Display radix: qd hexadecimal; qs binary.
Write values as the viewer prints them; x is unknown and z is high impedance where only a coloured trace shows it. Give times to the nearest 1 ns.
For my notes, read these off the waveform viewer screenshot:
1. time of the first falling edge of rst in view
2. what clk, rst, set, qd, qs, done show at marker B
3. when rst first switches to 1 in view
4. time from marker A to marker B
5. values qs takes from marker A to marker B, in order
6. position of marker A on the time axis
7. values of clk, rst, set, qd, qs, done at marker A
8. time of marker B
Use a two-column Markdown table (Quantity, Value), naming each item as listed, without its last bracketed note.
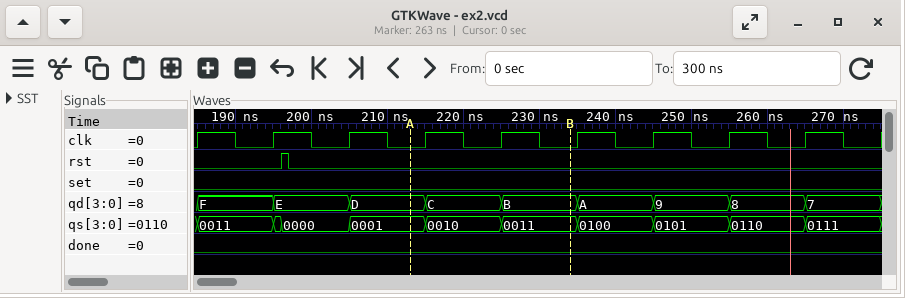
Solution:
| Quantity | Value |
|---|---|
| time of the first falling edge of rst in view | 197 ns |
| what clk, rst, set, qd, qs, done show at marker B | clk=0, rst=0, set=0, qd=B, qs=0011, done=0 |
| when rst first switches to 1 in view | 196 ns |
| time from marker A to marker B | 21 ns |
| values qs takes from marker A to marker B, in order | 0001, 0010, 0011 |
| position of marker A on the time axis | 213 ns |
| values of clk, rst, set, qd, qs, done at marker A | clk=0, rst=0, set=0, qd=D, qs=0001, done=0 |
| time of marker B | 234 ns |
